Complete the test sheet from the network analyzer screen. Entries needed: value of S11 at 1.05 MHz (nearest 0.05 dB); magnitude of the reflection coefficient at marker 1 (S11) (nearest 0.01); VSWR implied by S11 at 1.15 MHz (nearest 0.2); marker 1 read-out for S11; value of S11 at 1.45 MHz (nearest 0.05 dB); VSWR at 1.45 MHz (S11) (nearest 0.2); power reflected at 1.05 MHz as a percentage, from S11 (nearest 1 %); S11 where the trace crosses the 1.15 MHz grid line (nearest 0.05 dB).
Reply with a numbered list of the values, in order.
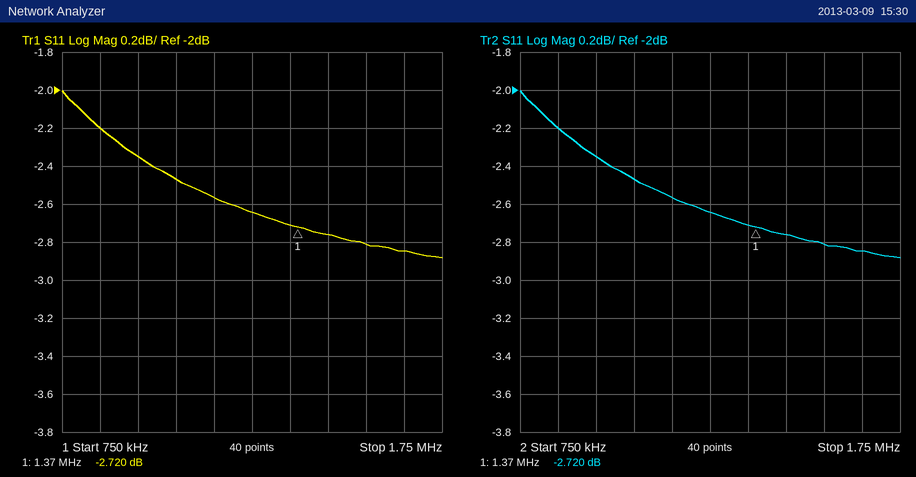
1. -2.45 dB
2. 0.73
3. 6.8
4. -2.720 dB
5. -2.75 dB
6. 6.4
7. 57 %
8. -2.55 dB
